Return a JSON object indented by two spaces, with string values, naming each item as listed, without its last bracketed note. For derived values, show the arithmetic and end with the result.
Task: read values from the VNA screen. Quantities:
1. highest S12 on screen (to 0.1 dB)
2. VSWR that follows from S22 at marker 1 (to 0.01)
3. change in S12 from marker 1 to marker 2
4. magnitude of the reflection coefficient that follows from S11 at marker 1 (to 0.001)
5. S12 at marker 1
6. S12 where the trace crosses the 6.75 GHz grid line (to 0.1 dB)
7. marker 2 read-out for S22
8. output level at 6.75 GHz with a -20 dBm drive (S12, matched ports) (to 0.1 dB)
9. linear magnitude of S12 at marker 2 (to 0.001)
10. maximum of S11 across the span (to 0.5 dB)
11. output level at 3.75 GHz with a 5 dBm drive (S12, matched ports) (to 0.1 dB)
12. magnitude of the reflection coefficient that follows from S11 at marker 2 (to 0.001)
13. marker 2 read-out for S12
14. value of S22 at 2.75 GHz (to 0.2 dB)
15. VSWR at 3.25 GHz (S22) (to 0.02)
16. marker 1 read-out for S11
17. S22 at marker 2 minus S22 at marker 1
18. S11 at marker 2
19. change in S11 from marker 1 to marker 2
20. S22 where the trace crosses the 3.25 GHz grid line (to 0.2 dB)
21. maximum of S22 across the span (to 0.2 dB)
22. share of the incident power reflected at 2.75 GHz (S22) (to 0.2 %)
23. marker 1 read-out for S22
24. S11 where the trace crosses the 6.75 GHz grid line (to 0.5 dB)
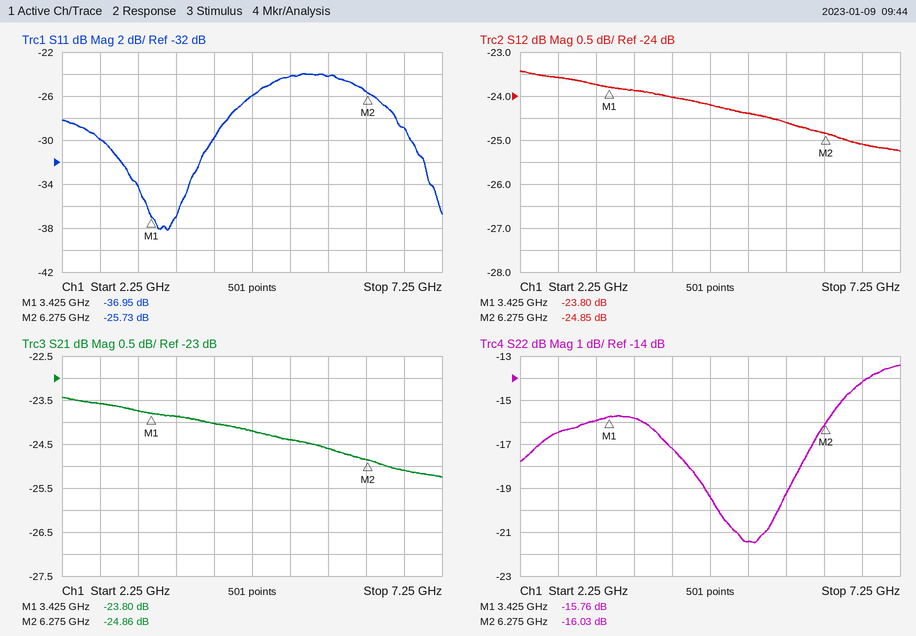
{
  "highest S12 on screen": "-23.4 dB",
  "VSWR that follows from S22 at marker 1": "(1 + 0.1629)/(1 − 0.1629) ≈ 1.39",
  "change in S12 from marker 1 to marker 2": "-24.85 − (-23.8) = -1.05 dB",
  "magnitude of the reflection coefficient that follows from S11 at marker 1": "10^(-36.95/20) ≈ 0.014",
  "S12 at marker 1": "-23.80 dB",
  "S12 where the trace crosses the 6.75 GHz grid line": "-25.1 dB",
  "marker 2 read-out for S22": "-16.03 dB",
  "output level at 6.75 GHz with a -20 dBm drive (S12, matched ports)": "-20 dBm + (-25.1 dB) = -45.1 dBm",
  "linear magnitude of S12 at marker 2": "10^(-24.85/20) ≈ 0.057",
  "maximum of S11 across the span": "-24.0 dB",
  "output level at 3.75 GHz with a 5 dBm drive (S12, matched ports)": "5 dBm + (-23.9 dB) = -18.9 dBm",
  "magnitude of the reflection coefficient that follows from S11 at marker 2": "10^(-25.73/20) ≈ 0.052",
  "marker 2 read-out for S12": "-24.85 dB",
  "value of S22 at 2.75 GHz": "-16.4 dB",
  "VSWR at 3.25 GHz (S22)": "|Γ| = 10^(-16/20) = 0.1585; VSWR = (1 + 0.1585)/(1 − 0.1585) ≈ 1.38",
  "marker 1 read-out for S11": "-36.95 dB",
  "S22 at marker 2 minus S22 at marker 1": "-16.03 − (-15.76) = -0.27 dB",
  "S11 at marker 2": "-25.73 dB",
  "change in S11 from marker 1 to marker 2": "-25.73 − (-36.95) = 11.22 dB",
  "S22 where the trace crosses the 3.25 GHz grid line": "-16.0 dB",
  "maximum of S22 across the span": "-13.4 dB",
  "share of the incident power reflected at 2.75 GHz (S22)": "10^(-16.4/10) ≈ 2.29 %, so 2.2 % to the nearest 0.2 %",
  "marker 1 read-out for S22": "-15.76 dB",
  "S11 where the trace crosses the 6.75 GHz grid line": "-29.0 dB"
}
